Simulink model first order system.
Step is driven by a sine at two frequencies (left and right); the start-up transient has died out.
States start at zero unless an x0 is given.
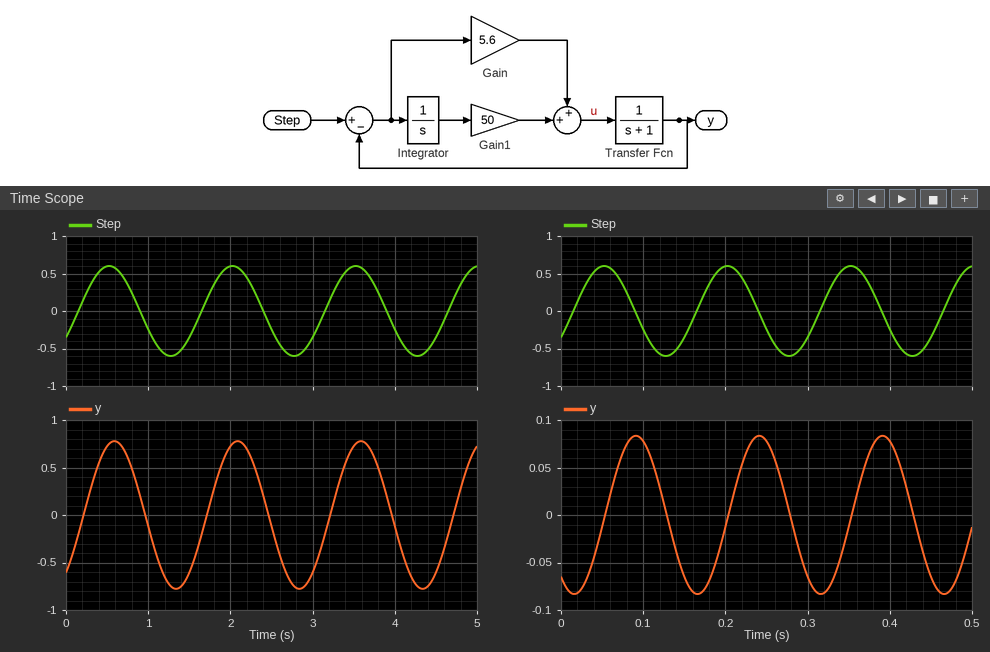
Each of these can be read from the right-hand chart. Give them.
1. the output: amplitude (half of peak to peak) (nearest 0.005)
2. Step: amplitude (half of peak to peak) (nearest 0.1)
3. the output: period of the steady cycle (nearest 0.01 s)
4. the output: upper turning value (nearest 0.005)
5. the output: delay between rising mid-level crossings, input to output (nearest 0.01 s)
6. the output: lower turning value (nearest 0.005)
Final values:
0.085
0.6
0.15 s
0.085
0.04 s
-0.085
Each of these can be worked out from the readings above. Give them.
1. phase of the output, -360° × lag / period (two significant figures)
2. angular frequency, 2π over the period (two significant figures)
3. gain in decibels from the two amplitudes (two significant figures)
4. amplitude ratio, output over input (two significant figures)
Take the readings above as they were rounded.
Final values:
-96°
42 rad/s
-17 dB
0.14
